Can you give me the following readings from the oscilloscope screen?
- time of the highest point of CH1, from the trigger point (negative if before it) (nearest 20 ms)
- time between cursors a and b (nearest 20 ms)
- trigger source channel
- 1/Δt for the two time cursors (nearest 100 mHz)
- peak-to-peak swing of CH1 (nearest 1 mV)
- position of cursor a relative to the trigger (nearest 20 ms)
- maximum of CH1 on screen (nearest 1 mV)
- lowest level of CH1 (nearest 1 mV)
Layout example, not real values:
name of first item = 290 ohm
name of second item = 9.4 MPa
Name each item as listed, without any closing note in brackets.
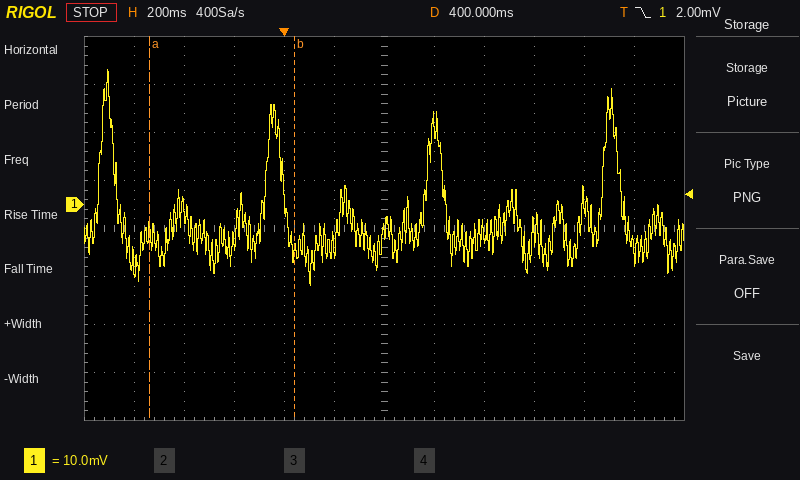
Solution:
time of the highest point of CH1, from the trigger point (negative if before it) = -700 ms
time between cursors a and b = 580 ms
trigger source channel = CH1
1/Δt for the two time cursors = 1.7 Hz
peak-to-peak swing of CH1 = 45 mV
position of cursor a relative to the trigger = -540 ms
maximum of CH1 on screen = 28 mV
lowest level of CH1 = -17 mV
